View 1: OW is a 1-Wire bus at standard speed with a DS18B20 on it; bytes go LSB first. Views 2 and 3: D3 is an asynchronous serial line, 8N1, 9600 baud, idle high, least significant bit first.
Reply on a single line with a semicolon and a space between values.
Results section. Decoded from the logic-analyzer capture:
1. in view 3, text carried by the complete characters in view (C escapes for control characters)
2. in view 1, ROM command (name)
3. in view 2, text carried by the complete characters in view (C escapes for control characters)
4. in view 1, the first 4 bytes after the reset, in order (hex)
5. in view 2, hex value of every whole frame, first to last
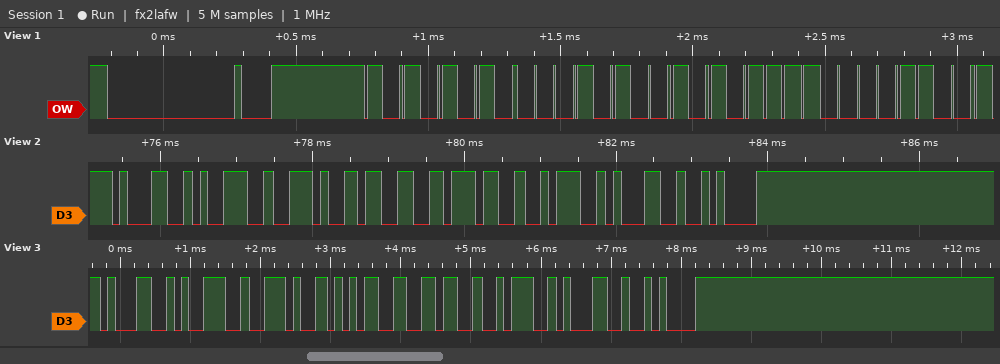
"19.56:1\n"; Match ROM; "19.37:1\n"; 55 28 F5 30; 31 39 2E 33 37 3A 31 0A
